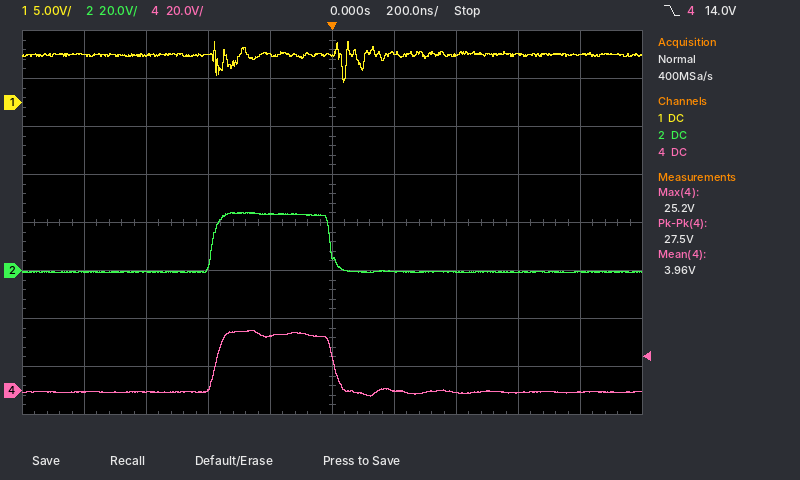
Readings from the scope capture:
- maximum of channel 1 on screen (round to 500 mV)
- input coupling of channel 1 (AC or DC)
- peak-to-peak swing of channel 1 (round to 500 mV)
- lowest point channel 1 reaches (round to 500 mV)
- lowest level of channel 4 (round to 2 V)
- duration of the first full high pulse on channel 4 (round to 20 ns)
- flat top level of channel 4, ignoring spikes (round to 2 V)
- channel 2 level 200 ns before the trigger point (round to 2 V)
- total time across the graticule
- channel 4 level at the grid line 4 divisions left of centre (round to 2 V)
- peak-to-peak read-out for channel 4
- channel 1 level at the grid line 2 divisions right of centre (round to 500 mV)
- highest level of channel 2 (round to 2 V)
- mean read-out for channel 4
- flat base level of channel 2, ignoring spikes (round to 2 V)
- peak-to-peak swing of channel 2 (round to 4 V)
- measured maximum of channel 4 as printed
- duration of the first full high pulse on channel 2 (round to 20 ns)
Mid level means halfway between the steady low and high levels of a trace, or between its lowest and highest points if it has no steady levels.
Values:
6.5 V
DC
4.5 V
2.0 V
-2 V
380 ns
24 V
24 V
2 µs
0 V
27.5 V
5.0 V
24 V
3.96 V
0 V
24 V
25.2 V
380 ns
